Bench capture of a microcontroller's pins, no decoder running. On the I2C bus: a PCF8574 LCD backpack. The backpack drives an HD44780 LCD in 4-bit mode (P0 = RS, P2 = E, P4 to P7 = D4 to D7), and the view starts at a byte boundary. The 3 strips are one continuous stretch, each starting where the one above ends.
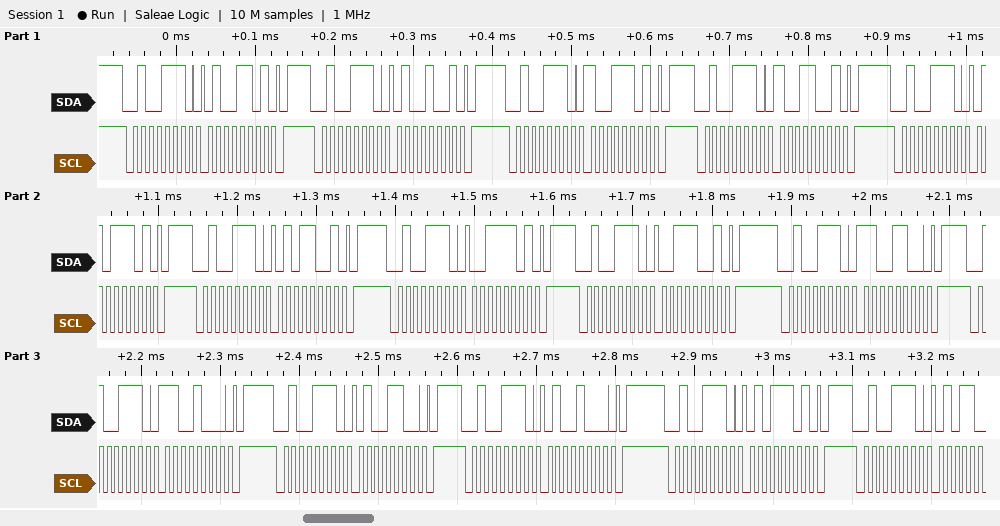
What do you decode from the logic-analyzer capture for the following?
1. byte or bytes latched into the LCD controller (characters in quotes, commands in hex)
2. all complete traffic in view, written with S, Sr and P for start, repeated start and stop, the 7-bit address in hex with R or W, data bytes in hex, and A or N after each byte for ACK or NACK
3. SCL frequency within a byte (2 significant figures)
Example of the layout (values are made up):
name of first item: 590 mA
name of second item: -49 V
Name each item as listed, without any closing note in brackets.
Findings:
byte or bytes latched into the LCD controller: 'I' 'S' 0xC4
all complete traffic in view, written with S, Sr and P for start, repeated start and stop, the 7-bit address in hex with R or W, data bytes in hex, and A or N after each byte for ACK or NACK: S 27W A 4D A P S 27W A 49 A P S 27W A 9D A P S 27W A 99 A P S 27W A 5D A P S 27W A 59 A P S 27W A 3D A P S 27W A 39 A P S 27W A CC A P S 27W A C8 A P S 27W A 4C A P S 27W A 48 A P S 27W A 5D A P S 27W A
SCL frequency within a byte: 100 kHz
